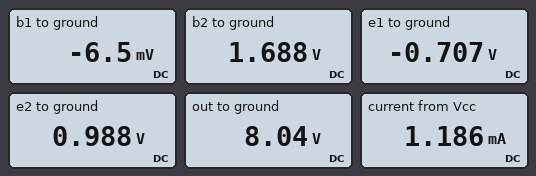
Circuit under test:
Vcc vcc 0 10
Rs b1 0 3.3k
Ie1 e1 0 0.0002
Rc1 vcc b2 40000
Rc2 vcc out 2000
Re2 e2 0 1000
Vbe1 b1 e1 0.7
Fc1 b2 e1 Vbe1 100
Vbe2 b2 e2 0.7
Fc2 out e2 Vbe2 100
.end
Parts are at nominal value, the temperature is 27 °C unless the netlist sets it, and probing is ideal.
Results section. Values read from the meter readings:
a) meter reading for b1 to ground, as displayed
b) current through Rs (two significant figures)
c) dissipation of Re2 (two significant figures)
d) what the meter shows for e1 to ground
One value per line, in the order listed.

-6.5 mV
2.0 µA
980 µW
-0.707 V
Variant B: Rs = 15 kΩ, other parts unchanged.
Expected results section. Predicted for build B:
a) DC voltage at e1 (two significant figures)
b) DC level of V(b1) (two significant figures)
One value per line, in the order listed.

-730 mV
-30 mV
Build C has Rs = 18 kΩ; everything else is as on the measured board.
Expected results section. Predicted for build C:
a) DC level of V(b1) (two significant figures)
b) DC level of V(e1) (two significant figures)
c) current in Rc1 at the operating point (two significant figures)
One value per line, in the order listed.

-36 mV
-740 mV
210 µA
